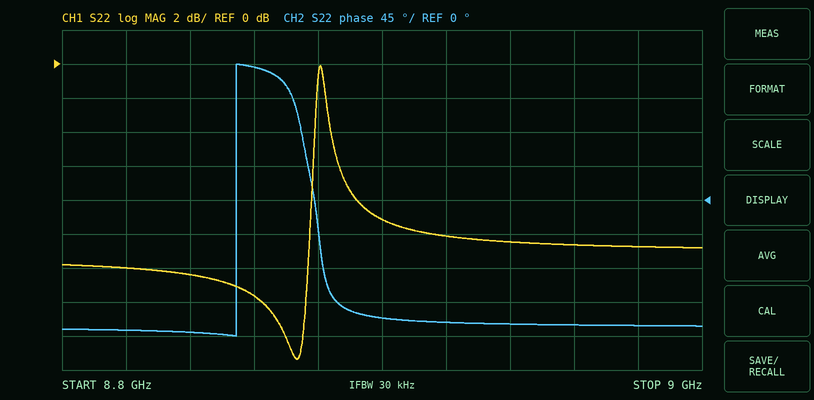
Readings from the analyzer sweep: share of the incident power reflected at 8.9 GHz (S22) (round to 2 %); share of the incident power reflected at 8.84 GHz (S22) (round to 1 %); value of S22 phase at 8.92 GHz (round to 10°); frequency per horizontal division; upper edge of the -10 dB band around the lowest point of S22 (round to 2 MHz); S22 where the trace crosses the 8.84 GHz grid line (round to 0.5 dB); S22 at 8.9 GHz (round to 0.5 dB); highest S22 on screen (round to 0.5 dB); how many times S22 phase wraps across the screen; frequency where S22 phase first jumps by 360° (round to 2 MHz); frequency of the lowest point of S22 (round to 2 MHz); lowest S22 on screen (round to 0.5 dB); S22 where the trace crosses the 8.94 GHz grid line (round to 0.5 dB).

12 %
6 %
-160°
20 MHz
8.878 GHz
-12.5 dB
-9.0 dB
0.0 dB
1
8.854 GHz
8.874 GHz
-17.5 dB
-10.5 dB
